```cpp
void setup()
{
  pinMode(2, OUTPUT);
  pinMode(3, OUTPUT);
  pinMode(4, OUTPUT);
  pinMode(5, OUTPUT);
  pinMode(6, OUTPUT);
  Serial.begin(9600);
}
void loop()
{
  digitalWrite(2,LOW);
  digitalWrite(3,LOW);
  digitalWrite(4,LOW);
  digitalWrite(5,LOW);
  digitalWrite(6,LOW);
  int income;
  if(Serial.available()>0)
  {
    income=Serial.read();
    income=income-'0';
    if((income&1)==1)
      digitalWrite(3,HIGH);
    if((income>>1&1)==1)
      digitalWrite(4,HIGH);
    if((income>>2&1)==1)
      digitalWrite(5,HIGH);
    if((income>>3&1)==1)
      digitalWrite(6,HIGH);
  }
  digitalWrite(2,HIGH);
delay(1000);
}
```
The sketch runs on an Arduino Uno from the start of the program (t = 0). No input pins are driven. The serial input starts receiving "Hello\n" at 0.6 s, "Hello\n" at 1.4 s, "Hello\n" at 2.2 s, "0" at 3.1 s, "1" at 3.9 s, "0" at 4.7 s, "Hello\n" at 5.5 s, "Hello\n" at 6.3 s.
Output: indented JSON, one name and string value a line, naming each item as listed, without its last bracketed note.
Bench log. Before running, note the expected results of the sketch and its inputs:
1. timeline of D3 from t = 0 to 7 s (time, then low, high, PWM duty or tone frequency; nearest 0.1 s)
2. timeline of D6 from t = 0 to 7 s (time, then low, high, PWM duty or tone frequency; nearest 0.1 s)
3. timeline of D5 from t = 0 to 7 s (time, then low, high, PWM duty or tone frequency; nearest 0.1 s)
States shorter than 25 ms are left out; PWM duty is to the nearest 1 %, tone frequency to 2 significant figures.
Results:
{
  "timeline of D3 from t = 0 to 7 s": "0 s low; 2 s high; 3 s low; 5 s high; 6 s low",
  "timeline of D6 from t = 0 to 7 s": "0 s low; 1 s high; 2 s low; 3 s high",
  "timeline of D5 from t = 0 to 7 s": "0 s low; 2 s high; 6 s low"
}
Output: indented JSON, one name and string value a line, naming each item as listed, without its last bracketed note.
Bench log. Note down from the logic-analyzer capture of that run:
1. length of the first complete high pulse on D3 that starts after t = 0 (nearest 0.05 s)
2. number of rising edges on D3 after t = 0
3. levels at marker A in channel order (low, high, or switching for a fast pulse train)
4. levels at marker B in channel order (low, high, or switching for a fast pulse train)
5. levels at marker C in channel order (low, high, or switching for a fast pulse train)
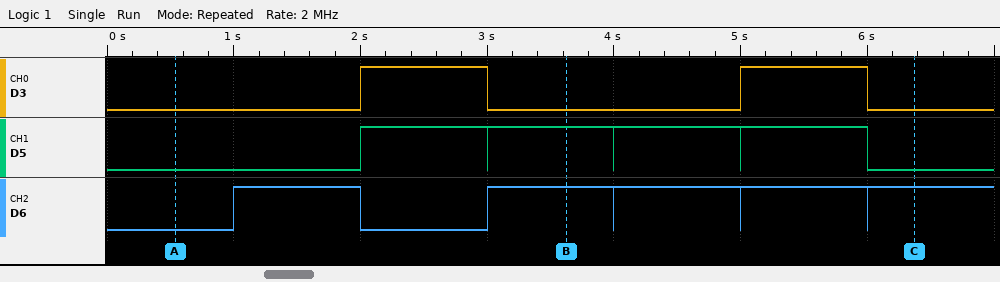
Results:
{
  "length of the first complete high pulse on D3 that starts after t = 0": "1.00 s",
  "number of rising edges on D3 after t = 0": "2",
  "levels at marker A in channel order": "D3 low, D5 low, D6 low",
  "levels at marker B in channel order": "D3 low, D5 high, D6 high",
  "levels at marker C in channel order": "D3 low, D5 low, D6 high"
}
